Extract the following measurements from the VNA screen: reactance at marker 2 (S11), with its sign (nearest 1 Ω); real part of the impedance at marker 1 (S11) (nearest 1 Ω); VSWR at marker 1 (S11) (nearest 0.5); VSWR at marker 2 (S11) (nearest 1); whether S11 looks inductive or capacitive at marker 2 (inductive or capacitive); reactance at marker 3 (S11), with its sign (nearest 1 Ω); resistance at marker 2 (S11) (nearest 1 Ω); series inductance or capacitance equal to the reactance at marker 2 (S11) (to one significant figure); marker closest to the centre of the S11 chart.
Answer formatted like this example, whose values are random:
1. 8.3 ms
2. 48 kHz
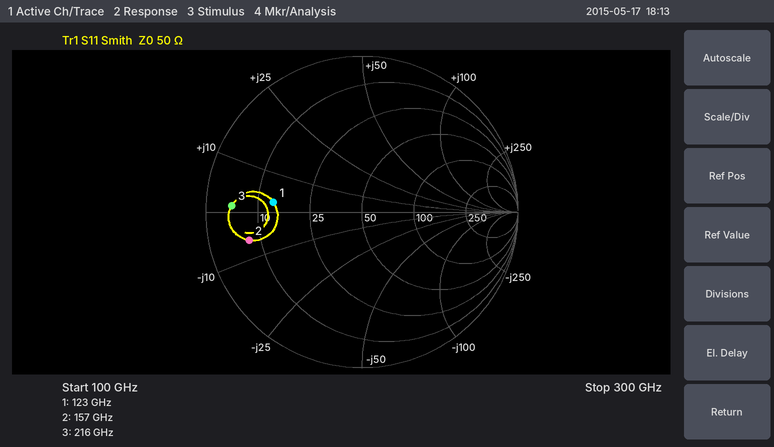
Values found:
1. -6 Ω
2. 14 Ω
3. 3.5
4. 7
5. capacitive
6. +1 Ω
7. 7 Ω
8. 200 fF
9. marker 1
